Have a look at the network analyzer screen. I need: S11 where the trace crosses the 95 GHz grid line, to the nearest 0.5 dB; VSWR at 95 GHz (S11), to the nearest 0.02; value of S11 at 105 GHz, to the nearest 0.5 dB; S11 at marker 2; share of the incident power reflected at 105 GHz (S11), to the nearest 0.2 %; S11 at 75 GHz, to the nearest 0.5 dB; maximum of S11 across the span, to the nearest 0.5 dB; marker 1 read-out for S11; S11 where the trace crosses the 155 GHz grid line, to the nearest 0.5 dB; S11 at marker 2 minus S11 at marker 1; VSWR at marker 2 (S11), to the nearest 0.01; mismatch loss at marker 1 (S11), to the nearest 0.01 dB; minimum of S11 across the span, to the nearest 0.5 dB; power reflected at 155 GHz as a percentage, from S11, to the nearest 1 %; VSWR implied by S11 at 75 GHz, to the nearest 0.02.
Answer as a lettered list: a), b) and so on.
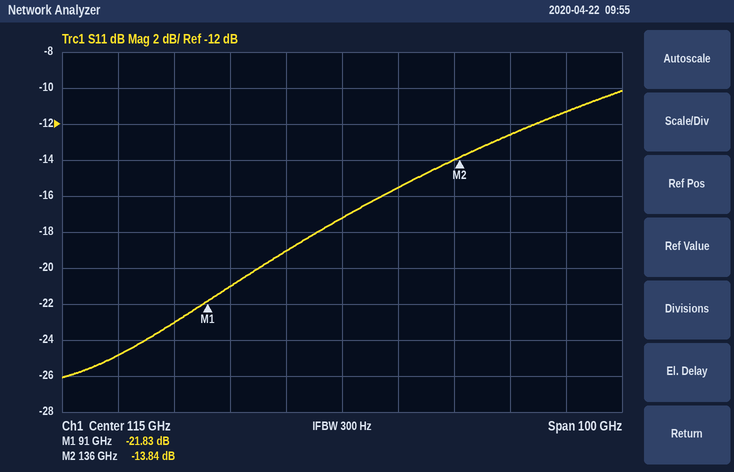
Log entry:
a) -21.0 dB
b) 1.20
c) -19.0 dB
d) -13.84 dB
e) 1.2 %
f) -25.0 dB
g) -10.0 dB
h) -21.83 dB
i) -11.5 dB
j) 7.99 dB
k) 1.51
l) 0.03 dB
m) -26.0 dB
n) 7 %
o) 1.12
